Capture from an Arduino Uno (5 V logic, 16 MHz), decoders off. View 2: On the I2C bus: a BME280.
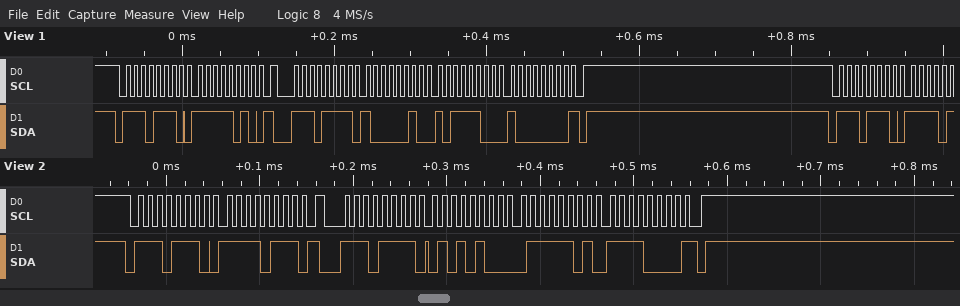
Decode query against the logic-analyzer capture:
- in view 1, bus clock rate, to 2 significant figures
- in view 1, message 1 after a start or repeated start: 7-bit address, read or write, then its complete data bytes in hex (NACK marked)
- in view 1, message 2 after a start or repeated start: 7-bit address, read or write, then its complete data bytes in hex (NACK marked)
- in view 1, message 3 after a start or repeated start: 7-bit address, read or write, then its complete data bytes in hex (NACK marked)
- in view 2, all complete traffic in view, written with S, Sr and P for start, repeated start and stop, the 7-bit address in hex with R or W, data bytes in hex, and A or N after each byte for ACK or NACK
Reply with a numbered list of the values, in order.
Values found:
1. 100 kHz
2. 0x77 write: FA
3. 0x77 read: 82 BC 80 NACK
4. 0x77 write
5. S 77W A F7 A Sr 77R A 54 A 7D A F0 N P
